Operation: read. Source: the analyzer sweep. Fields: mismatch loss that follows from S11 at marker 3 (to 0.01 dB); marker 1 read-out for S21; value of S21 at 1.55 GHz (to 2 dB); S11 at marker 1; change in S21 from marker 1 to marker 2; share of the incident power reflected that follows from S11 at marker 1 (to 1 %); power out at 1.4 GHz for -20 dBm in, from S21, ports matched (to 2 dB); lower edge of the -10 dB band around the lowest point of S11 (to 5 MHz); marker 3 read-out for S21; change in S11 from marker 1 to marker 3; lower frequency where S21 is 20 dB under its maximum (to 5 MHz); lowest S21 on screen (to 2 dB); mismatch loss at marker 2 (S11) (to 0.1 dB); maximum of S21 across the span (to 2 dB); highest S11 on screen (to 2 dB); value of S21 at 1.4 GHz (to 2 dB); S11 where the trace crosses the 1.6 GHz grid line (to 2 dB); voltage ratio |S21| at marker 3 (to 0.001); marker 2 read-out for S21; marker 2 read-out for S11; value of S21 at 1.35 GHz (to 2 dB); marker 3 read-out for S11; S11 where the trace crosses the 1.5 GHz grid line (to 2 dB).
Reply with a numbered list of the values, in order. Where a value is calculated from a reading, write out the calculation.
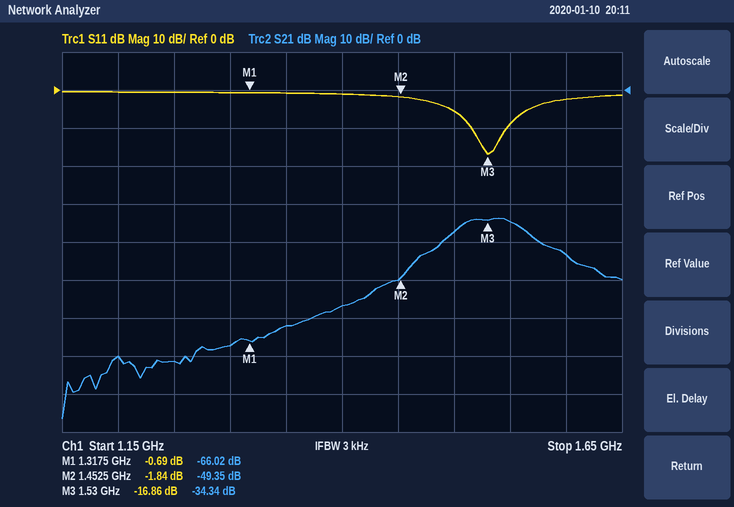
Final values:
1. −10 log10(1 − 10^(-16.86/10)) ≈ 0.09 dB
2. -66.02 dB
3. -34 dB
4. -0.69 dB
5. -49.35 − (-66.02) = 16.67 dB
6. 10^(-0.69/10) ≈ 85 %
7. -20 dBm + (-56 dB) = -76 dBm
8. 1.515 GHz
9. -34.34 dB
10. -16.86 − (-0.69) = -16.17 dB
11. 1.425 GHz
12. -86 dB
13. −10 log10(1 − 10^(-1.84/10)) ≈ 4.6 dB
14. -34 dB
15. 0 dB
16. -56 dB
17. -2 dB
18. 10^(-34.34/20) ≈ 0.019
19. -49.35 dB
20. -1.84 dB
21. -62 dB
22. -16.86 dB
23. -6 dB
